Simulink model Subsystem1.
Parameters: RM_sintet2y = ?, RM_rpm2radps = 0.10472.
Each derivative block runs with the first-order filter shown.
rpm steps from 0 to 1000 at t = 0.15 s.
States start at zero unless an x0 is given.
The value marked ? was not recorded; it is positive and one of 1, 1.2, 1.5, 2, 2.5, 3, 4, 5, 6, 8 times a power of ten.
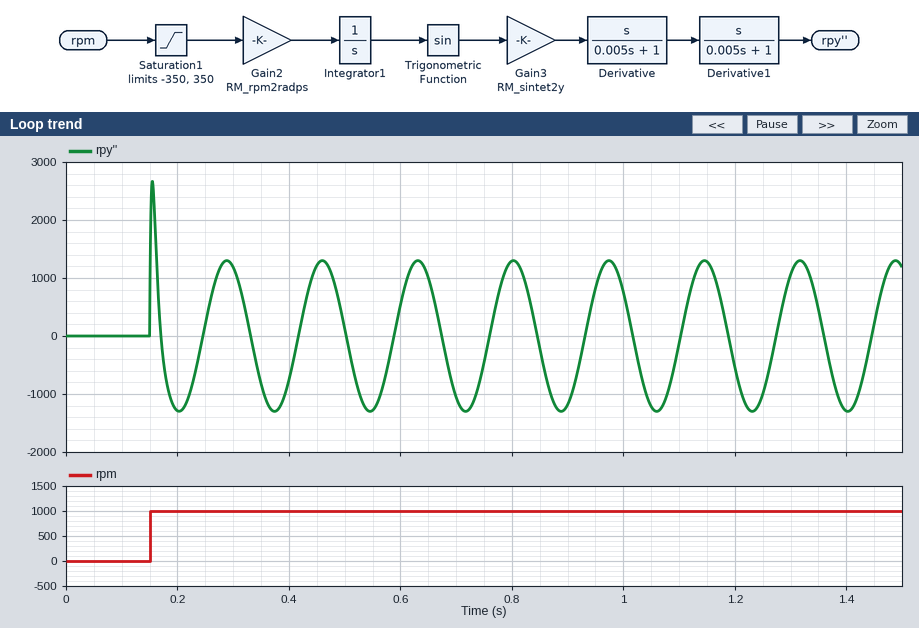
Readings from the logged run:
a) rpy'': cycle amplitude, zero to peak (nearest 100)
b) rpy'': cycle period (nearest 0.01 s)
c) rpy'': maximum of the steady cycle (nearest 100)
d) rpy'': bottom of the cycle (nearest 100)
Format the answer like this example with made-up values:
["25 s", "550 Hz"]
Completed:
["1300", "0.17 s", "1300", "-1300"]
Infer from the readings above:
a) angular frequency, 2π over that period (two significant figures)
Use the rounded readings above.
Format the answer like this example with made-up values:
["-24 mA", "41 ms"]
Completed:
["37 rad/s"]
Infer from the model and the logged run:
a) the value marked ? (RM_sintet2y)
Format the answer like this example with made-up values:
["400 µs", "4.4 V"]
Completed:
["1"]
